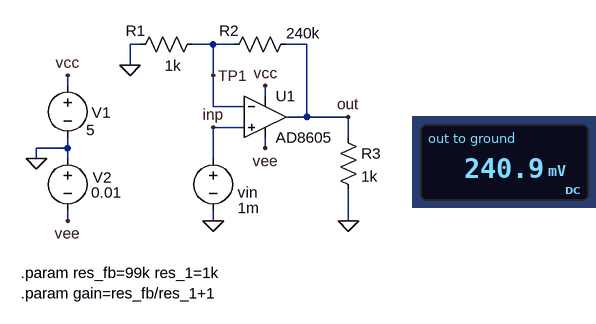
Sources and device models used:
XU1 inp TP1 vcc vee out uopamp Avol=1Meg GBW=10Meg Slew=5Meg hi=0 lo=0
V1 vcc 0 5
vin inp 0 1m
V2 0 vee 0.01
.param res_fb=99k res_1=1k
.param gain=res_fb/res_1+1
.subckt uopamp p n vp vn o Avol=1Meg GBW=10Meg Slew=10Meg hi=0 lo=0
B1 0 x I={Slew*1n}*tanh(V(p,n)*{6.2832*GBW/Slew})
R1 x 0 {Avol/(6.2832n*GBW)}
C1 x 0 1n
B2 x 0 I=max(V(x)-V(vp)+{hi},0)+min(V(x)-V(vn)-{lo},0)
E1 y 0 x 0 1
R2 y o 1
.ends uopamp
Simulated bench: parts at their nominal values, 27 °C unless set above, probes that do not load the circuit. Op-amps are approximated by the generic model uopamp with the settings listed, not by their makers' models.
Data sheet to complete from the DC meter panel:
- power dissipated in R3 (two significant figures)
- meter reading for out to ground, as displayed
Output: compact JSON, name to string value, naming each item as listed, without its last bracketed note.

{"power dissipated in R3": "58 µW", "meter reading for out to ground, as displayed": "240.9 mV"}
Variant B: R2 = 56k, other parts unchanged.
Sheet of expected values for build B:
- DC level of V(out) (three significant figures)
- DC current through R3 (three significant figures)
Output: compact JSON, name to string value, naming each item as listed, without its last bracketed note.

{"DC level of V(out)": "57.0 mV", "DC current through R3": "57.0 µA"}
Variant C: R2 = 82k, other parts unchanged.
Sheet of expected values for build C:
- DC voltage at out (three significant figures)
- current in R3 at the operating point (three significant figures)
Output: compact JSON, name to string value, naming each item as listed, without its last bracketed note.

{"DC voltage at out": "83.0 mV", "current in R3 at the operating point": "83.0 µA"}
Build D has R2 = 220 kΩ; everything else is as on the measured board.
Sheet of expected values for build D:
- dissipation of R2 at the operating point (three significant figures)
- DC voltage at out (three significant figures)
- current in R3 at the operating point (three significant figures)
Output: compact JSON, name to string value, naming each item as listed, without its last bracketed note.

{"dissipation of R2 at the operating point": "220 nW", "DC voltage at out": "221 mV", "current in R3 at the operating point": "221 µA"}
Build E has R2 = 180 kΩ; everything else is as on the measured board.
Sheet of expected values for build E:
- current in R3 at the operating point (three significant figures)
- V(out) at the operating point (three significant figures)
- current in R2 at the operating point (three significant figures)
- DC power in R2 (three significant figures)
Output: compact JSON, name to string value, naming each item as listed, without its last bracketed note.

{"current in R3 at the operating point": "181 µA", "V(out) at the operating point": "181 mV", "current in R2 at the operating point": "1.00 µA", "DC power in R2": "180 nW"}
